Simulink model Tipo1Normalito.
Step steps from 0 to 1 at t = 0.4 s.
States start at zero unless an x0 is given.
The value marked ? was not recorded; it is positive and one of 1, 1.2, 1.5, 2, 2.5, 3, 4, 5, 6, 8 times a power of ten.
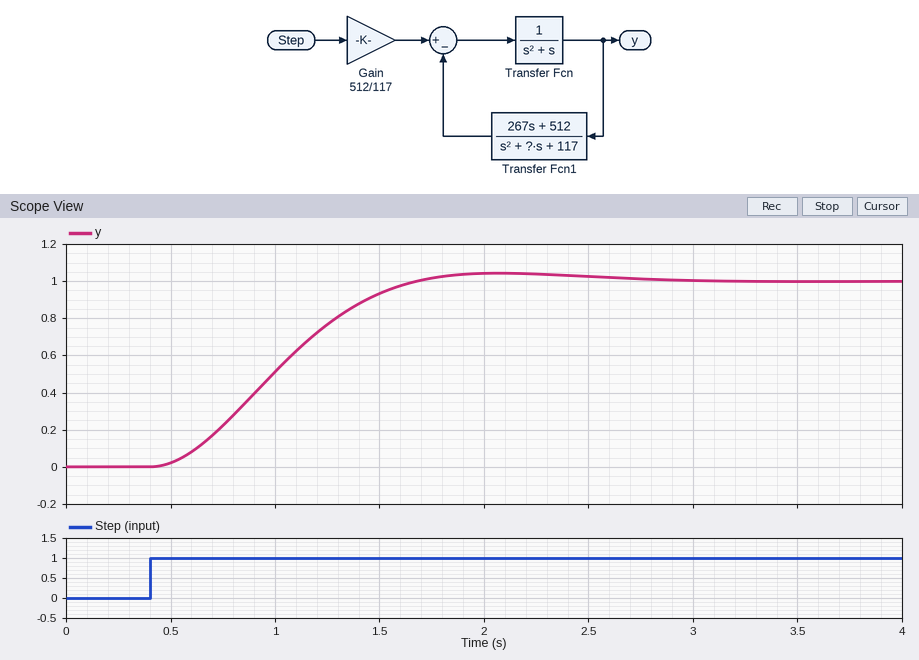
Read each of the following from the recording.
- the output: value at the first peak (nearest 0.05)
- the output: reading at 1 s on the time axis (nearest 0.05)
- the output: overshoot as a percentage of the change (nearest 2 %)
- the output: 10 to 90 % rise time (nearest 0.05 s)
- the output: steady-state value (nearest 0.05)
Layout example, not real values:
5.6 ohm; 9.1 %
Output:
1.05; 0.50; 4 %; 0.80 s; 1.00
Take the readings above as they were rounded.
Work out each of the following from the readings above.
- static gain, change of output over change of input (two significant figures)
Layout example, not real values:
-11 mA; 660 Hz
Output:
1.0
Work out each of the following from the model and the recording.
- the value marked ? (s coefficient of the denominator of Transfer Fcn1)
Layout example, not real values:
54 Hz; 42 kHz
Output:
20
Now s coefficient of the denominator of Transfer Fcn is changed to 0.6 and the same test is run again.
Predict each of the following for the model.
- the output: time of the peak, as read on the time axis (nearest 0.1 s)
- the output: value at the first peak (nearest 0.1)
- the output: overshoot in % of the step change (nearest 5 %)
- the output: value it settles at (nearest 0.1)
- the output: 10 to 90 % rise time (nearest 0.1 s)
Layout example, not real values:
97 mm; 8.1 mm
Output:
1.9 s; 1.1; 10 %; 1.0; 0.7 s
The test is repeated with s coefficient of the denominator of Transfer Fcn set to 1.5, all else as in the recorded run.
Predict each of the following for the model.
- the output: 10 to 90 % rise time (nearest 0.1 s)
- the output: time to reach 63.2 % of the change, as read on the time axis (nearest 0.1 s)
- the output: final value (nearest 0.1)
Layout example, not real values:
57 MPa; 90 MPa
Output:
1.0 s; 1.2 s; 1.0
